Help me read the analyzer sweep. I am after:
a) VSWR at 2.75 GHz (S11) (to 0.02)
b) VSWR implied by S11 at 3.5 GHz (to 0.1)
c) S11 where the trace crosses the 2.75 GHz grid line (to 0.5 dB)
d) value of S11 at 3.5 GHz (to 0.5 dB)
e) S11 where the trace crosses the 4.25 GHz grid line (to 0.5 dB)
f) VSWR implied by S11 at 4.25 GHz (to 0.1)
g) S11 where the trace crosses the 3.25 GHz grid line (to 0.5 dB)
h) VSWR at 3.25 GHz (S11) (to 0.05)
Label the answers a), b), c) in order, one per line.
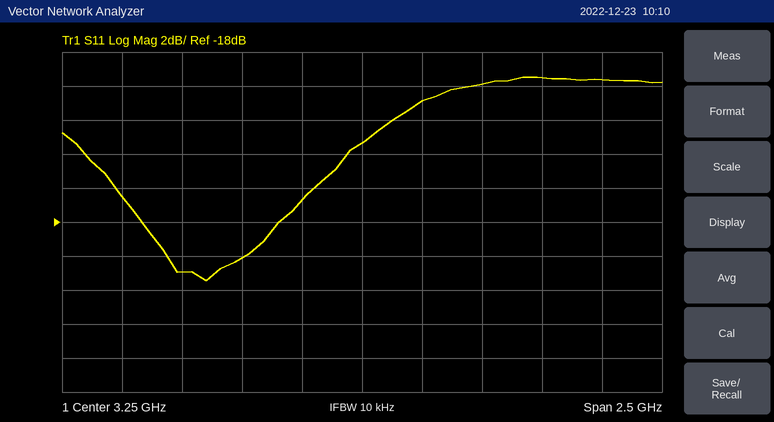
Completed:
a) 1.22
b) 1.8
c) -20.0 dB
d) -11.0 dB
e) -9.5 dB
f) 2.0
g) -13.5 dB
h) 1.55
